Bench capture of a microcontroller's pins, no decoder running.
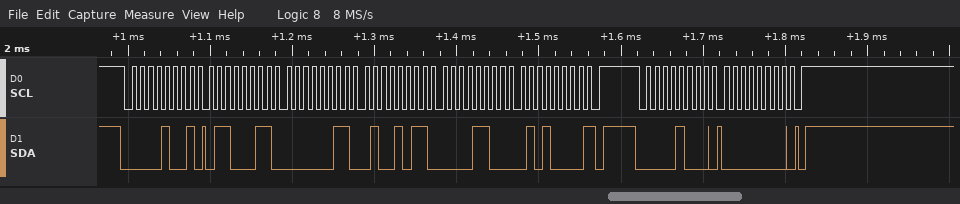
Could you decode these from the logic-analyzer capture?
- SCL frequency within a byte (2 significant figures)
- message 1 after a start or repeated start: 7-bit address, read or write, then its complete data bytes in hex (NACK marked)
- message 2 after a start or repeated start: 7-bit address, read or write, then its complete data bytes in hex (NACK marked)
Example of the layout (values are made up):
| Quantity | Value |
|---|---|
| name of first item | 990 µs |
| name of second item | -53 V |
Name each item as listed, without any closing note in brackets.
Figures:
| Quantity | Value |
|---|---|
| SCL frequency within a byte | 100 kHz |
| message 1 after a start or repeated start: 7-bit address, read or write, then its complete data bytes in hex | 0x04 read: 63 03 4B 0C 50 NACK |
| message 2 after a start or repeated start: 7-bit address, read or write, then its complete data bytes in hex | 0x04 write: 00 |
